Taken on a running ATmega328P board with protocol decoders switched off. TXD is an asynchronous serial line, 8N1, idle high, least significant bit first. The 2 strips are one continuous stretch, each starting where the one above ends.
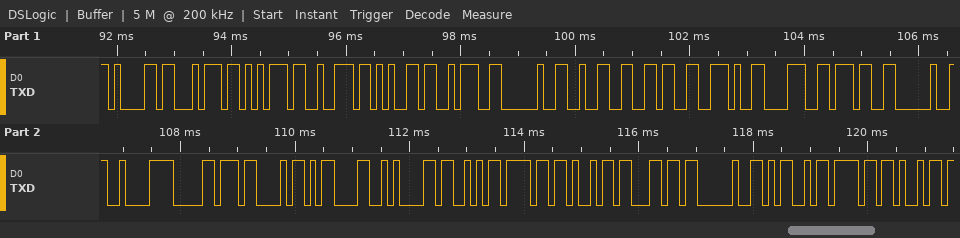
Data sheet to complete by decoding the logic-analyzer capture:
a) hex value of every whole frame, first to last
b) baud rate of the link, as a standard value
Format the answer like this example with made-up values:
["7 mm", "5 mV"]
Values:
["61 74 75 72 65 3A 20 32 36 2E 38 37 20 C2 B0 43 0D 0A 53 6F 69 6C 20 4D 6F 69", "9600 baud"]
